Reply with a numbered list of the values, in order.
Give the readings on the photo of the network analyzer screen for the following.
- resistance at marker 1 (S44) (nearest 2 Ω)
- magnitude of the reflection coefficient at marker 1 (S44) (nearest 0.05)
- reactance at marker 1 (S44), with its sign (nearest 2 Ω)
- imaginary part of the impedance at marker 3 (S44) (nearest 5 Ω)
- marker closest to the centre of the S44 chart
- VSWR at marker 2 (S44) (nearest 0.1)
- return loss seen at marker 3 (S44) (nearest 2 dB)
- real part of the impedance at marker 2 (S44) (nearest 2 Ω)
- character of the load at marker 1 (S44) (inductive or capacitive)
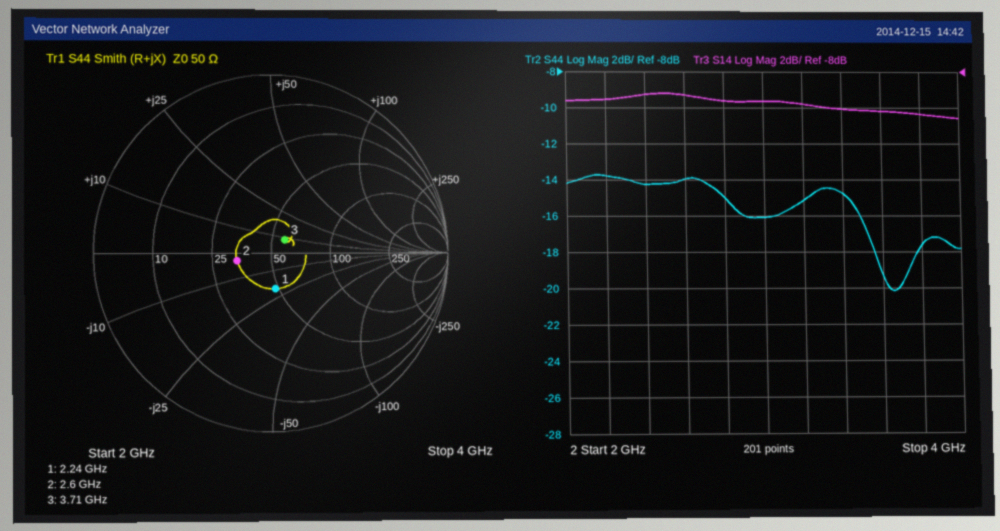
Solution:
1. 48 Ω
2. 0.20
3. -20 Ω
4. +10 Ω
5. marker 3
6. 1.5
7. 20 dB
8. 34 Ω
9. capacitive
